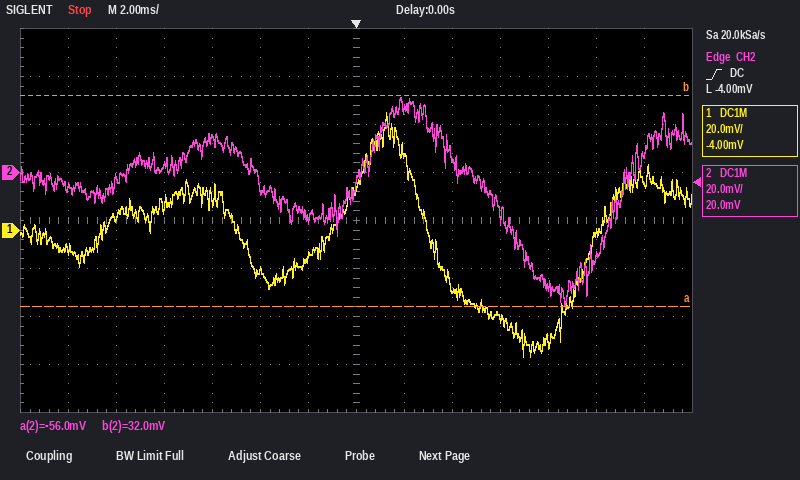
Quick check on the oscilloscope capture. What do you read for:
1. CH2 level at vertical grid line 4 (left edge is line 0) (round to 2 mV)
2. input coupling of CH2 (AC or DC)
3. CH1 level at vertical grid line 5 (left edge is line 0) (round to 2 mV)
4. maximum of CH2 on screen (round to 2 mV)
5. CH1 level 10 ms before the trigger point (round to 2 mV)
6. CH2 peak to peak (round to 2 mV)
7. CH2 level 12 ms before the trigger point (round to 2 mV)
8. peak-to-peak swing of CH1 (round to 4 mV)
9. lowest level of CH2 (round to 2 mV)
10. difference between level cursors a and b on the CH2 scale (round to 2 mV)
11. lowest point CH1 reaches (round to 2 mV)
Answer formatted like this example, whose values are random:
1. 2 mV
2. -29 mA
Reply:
1. 14 mV
2. DC
3. -16 mV
4. 32 mV
5. 6 mV
6. 88 mV
7. -6 mV
8. 100 mV
9. -56 mV
10. 88 mV
11. -52 mV
